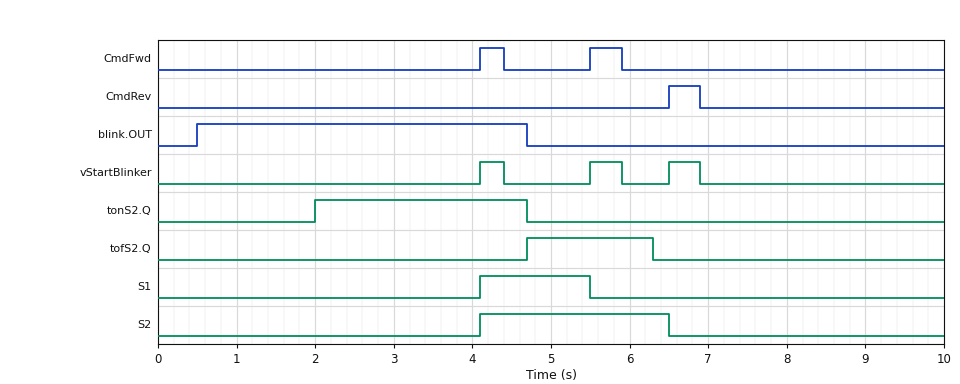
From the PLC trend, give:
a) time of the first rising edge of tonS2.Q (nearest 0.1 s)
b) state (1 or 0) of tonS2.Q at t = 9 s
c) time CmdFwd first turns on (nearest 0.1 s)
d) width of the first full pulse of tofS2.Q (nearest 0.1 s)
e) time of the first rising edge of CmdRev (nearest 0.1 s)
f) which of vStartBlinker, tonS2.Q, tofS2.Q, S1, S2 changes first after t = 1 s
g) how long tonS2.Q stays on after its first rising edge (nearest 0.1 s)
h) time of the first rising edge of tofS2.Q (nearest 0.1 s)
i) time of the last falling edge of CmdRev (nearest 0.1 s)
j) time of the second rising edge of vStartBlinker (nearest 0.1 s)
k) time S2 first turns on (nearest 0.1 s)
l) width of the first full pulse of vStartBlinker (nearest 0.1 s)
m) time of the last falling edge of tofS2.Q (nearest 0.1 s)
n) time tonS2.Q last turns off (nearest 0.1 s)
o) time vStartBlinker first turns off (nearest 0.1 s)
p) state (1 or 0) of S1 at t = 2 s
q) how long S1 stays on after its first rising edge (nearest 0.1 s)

2.0 s
0
4.1 s
1.6 s
6.5 s
tonS2.Q
2.7 s
4.7 s
6.9 s
5.5 s
4.1 s
0.3 s
6.3 s
4.7 s
4.4 s
0
1.4 s
